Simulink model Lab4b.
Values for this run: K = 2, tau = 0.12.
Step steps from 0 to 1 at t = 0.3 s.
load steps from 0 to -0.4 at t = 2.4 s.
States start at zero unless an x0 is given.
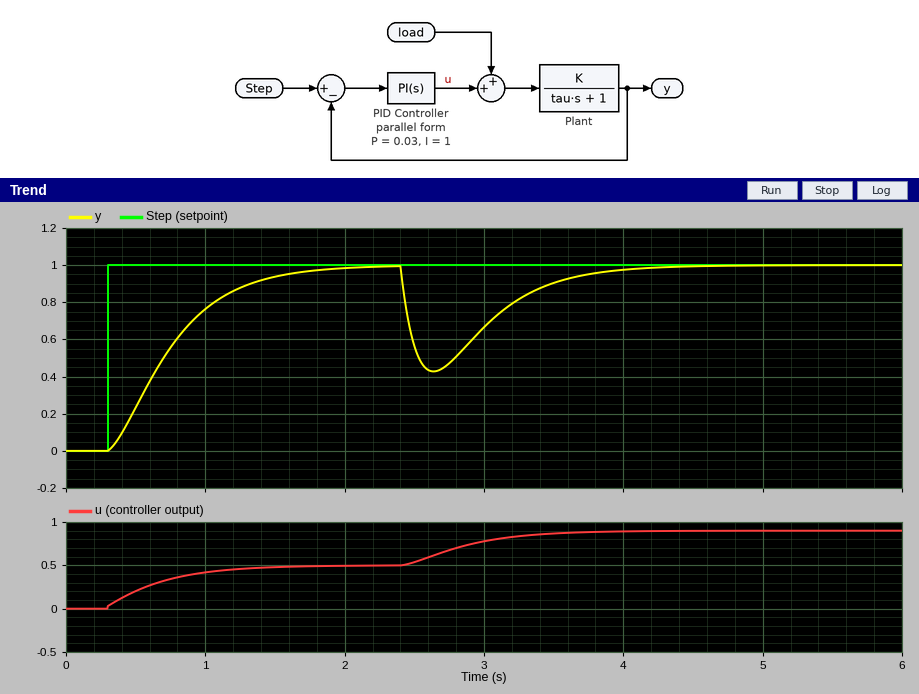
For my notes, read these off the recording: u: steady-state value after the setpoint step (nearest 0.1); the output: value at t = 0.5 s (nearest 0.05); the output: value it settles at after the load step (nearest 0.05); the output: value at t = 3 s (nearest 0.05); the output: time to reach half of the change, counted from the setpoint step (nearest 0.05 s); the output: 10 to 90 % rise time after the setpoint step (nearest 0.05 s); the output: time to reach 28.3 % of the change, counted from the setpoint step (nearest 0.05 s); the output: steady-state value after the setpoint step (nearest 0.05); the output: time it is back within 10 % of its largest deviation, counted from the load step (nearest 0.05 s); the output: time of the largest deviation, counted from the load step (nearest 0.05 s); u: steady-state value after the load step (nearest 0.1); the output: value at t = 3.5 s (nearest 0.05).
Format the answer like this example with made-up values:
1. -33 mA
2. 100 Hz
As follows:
1. 0.5
2. 0.25
3. 1.00
4. 0.65
5. 0.40 s
6. 0.90 s
7. 0.25 s
8. 1.00
9. 1.30 s
10. 0.25 s
11. 0.9
12. 0.90
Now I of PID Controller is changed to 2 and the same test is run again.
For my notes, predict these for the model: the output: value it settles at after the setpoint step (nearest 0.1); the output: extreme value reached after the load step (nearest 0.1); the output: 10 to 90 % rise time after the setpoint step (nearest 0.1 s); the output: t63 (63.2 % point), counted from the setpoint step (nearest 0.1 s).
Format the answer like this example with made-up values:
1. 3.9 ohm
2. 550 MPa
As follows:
1. 1.0
2. 0.5
3. 0.4 s
4. 0.3 s
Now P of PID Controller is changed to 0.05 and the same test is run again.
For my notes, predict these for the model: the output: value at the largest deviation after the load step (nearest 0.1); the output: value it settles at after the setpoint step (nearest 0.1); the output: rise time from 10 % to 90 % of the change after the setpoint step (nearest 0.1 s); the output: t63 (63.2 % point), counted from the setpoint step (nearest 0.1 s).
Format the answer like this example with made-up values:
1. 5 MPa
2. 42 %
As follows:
1. 0.4
2. 1.0
3. 1.0 s
4. 0.5 s
